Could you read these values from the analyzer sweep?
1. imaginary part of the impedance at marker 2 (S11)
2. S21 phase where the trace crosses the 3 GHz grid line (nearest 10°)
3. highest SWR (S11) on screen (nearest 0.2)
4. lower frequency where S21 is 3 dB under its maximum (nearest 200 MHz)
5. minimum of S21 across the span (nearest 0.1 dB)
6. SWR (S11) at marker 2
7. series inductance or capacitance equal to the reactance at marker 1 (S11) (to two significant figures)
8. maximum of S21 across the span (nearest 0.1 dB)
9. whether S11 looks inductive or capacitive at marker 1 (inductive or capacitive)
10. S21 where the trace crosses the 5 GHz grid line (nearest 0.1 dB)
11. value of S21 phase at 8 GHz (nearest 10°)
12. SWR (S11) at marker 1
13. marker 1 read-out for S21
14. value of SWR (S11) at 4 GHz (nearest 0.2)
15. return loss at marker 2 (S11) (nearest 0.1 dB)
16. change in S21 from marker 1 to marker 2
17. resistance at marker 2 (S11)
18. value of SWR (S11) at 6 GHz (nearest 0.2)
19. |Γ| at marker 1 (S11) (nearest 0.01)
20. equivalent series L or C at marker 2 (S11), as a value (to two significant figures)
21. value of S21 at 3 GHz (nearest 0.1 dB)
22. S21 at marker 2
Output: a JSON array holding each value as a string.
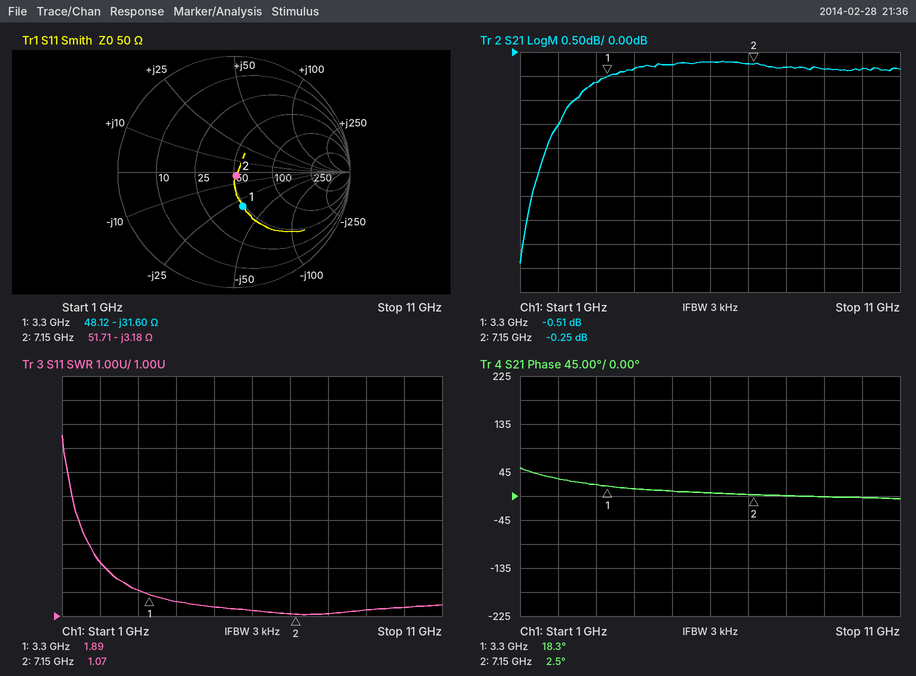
["-3.18 Ω", "20°", "8.6", "1.2 GHz", "-4.4 dB", "1.07", "1.5 pF", "-0.2 dB", "capacitive", "-0.3 dB", "0°", "1.89", "-0.51 dB", "1.6", "29.0 dB", "0.26 dB", "51.71 Ω", "1.2", "0.31", "7.0 pF", "-0.6 dB", "-0.25 dB"]
